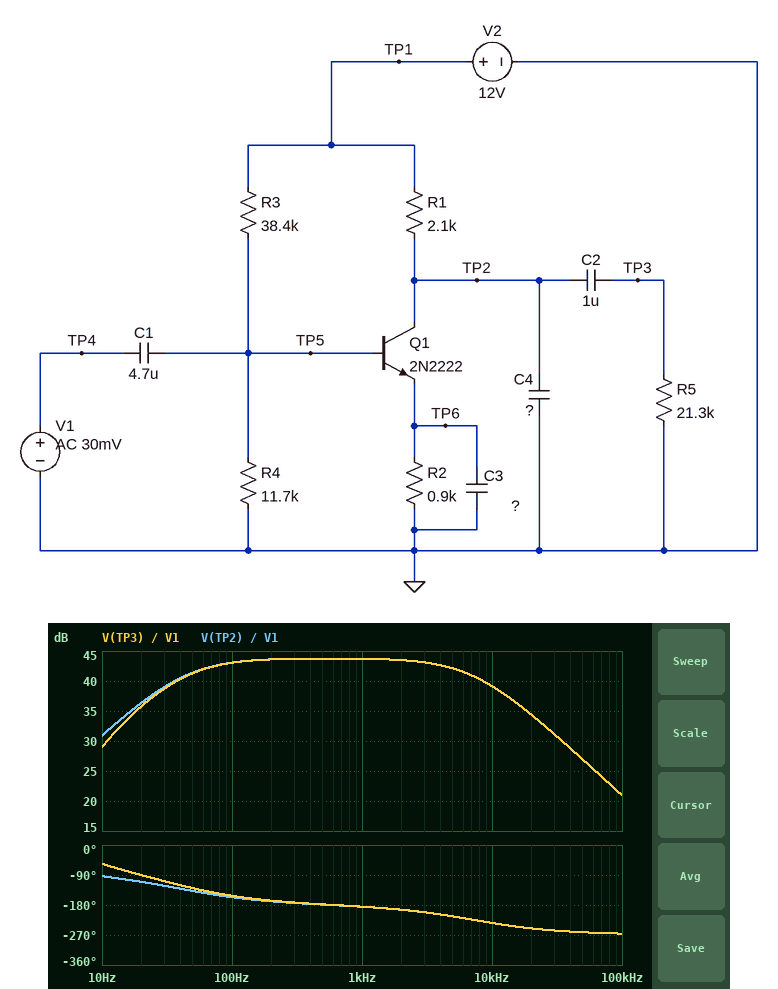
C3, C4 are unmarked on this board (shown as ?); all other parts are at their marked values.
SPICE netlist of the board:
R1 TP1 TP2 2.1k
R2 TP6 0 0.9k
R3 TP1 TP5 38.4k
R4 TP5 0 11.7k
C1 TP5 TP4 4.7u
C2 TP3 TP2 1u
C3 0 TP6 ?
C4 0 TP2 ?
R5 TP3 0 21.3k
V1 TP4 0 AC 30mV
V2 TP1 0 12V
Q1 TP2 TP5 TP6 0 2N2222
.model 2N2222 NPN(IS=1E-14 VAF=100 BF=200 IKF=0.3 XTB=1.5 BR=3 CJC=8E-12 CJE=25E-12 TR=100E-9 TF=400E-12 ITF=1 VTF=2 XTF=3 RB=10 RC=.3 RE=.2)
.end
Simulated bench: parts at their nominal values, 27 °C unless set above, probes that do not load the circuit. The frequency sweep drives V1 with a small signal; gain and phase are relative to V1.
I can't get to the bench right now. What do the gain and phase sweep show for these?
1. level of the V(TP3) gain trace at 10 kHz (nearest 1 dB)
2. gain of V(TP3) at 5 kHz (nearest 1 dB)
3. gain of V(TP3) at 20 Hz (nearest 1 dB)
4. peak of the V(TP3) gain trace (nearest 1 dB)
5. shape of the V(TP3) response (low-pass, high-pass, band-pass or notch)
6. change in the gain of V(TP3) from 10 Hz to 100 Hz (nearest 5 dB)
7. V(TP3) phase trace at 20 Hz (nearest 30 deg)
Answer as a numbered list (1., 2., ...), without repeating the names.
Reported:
1. 39 dB
2. 42 dB
3. 36 dB
4. 44 dB
5. band-pass
6. 15 dB
7. -90 deg
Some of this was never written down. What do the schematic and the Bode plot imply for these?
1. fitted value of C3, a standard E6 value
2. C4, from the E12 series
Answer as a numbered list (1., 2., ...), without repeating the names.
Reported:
1. 470 µF
2. 12 nF
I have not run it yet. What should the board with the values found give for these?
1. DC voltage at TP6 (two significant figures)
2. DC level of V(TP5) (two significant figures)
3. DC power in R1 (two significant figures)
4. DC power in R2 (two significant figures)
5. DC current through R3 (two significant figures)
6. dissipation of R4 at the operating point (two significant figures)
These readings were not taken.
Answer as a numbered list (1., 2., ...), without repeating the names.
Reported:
1. 2.0 V
2. 2.7 V
3. 11 mW
4. 4.6 mW
5. 240 µA
6. 630 µW
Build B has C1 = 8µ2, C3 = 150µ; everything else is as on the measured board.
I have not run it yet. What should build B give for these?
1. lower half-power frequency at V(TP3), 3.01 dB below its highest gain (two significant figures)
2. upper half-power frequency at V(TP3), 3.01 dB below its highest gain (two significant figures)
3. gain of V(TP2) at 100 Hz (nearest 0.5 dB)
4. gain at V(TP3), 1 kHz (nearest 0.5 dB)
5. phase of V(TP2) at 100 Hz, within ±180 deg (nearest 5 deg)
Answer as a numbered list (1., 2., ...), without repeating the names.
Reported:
1. 94 Hz
2. 7.4 kHz
3. 41.0 dB
4. 43.5 dB
5. -135 deg
